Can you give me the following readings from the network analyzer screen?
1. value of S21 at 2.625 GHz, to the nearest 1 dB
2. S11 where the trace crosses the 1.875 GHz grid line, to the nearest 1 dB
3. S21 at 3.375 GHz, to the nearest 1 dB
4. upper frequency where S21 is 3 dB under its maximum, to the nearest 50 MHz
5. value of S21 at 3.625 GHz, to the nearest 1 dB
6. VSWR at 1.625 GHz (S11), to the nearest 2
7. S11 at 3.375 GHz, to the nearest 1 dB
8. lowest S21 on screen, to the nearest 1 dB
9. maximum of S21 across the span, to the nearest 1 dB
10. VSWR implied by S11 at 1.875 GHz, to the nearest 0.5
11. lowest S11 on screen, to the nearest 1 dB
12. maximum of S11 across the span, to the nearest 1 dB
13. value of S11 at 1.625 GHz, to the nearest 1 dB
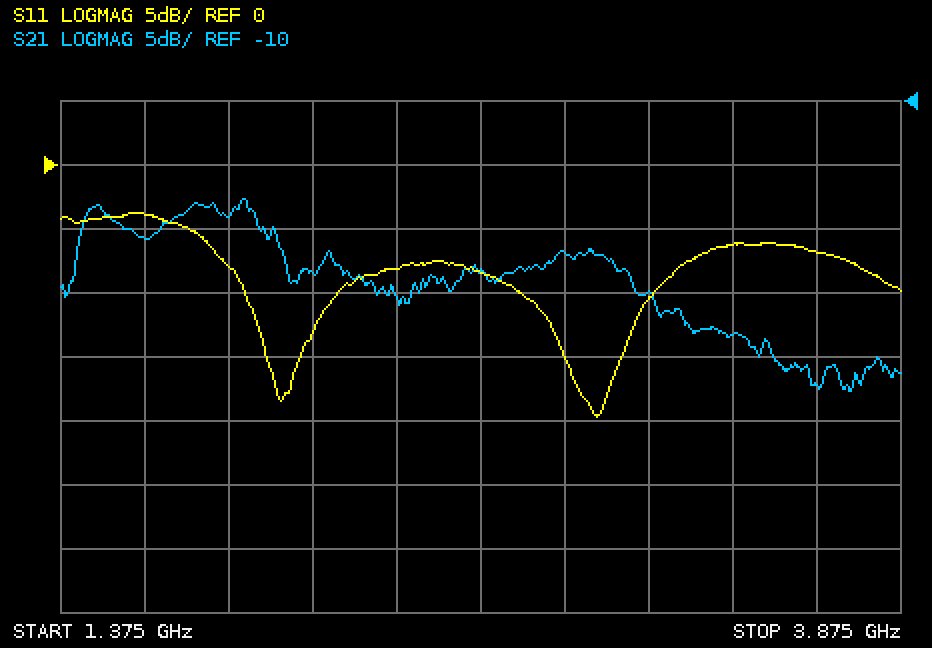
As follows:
-23 dB
-8 dB
-28 dB
2.00 GHz
-32 dB
4
-6 dB
-33 dB
-18 dB
2.5
-20 dB
-4 dB
-4 dB
